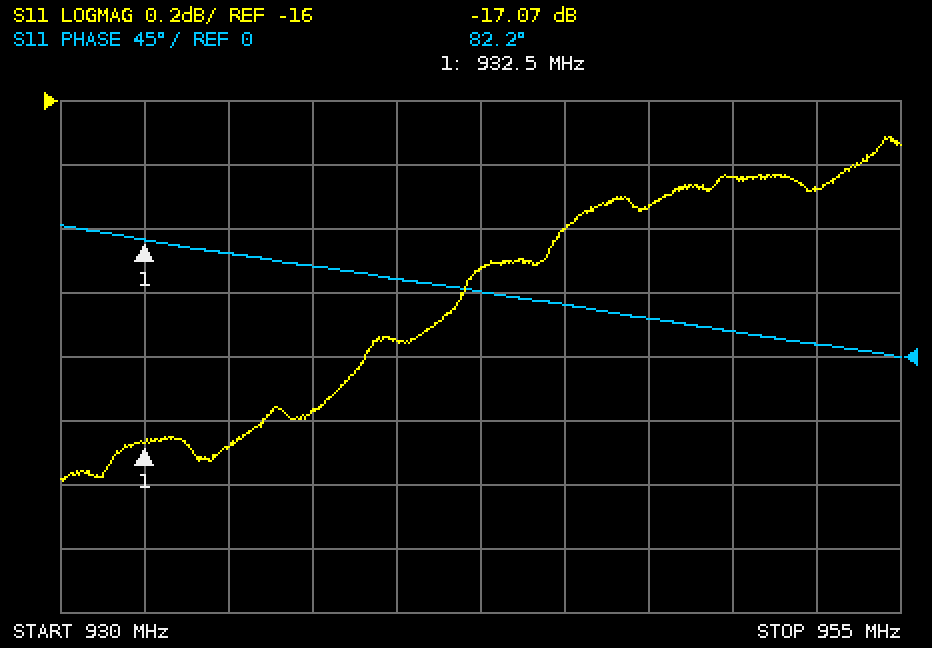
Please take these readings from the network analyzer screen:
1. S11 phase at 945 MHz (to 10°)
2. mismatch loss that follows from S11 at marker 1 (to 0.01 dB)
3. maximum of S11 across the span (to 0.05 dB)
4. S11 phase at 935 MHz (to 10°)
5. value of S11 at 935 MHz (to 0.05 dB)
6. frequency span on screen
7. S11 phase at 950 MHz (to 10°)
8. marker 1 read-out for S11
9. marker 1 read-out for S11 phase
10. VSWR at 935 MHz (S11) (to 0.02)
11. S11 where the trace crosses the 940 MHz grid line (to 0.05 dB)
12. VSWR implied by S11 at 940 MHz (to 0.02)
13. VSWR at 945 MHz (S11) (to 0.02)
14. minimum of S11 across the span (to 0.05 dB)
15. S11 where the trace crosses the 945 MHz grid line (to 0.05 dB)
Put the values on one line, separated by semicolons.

40°; 0.09 dB; -16.10 dB; 70°; -17.10 dB; 25 MHz; 20°; -17.07 dB; 82.2°; 1.32; -16.75 dB; 1.34; 1.36; -17.20 dB; -16.40 dB
